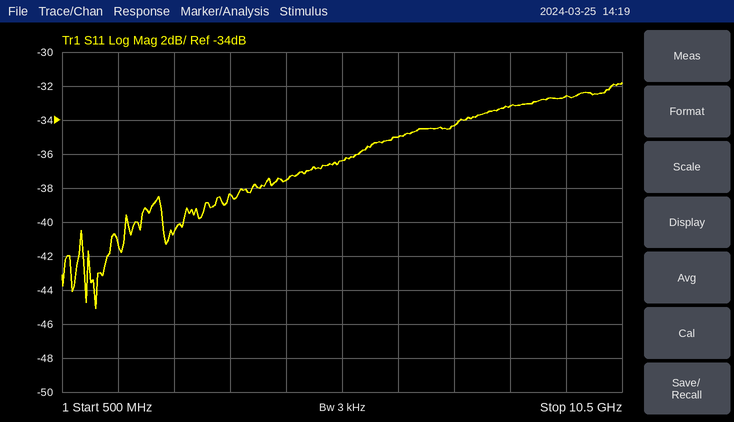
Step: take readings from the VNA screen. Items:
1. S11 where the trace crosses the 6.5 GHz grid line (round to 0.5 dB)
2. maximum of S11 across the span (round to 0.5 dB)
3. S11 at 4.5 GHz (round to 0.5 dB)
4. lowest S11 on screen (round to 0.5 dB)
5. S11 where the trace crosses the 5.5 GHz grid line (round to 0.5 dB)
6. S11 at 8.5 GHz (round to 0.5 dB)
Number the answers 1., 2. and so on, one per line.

1. -35.0 dB
2. -32.0 dB
3. -37.5 dB
4. -45.0 dB
5. -36.5 dB
6. -33.0 dB
